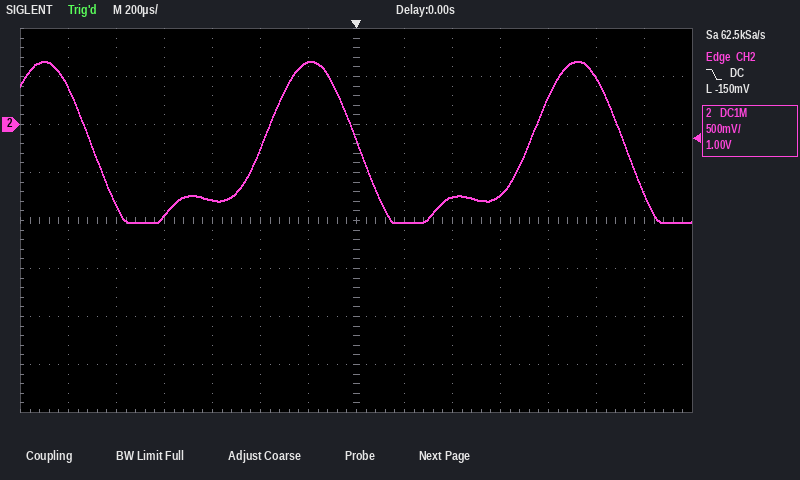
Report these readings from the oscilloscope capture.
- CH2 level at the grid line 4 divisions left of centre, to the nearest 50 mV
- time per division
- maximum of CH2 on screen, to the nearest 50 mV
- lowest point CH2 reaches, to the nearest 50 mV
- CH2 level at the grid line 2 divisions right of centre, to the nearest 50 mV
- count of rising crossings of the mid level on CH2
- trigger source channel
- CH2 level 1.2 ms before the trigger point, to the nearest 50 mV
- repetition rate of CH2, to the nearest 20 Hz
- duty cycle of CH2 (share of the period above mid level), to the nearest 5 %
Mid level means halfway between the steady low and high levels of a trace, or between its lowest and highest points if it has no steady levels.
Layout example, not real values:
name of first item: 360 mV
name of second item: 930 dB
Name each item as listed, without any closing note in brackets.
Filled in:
CH2 level at the grid line 4 divisions left of centre, to the nearest 50 mV: -950 mV
time per division: 200 µs
maximum of CH2 on screen, to the nearest 50 mV: 650 mV
lowest point CH2 reaches, to the nearest 50 mV: -1.00 V
CH2 level at the grid line 2 divisions right of centre, to the nearest 50 mV: -750 mV
count of rising crossings of the mid level on CH2: 2
trigger source channel: CH2
CH2 level 1.2 ms before the trigger point, to the nearest 50 mV: 400 mV
repetition rate of CH2, to the nearest 20 Hz: 900 Hz
duty cycle of CH2 (share of the period above mid level), to the nearest 5 %: 35 %
